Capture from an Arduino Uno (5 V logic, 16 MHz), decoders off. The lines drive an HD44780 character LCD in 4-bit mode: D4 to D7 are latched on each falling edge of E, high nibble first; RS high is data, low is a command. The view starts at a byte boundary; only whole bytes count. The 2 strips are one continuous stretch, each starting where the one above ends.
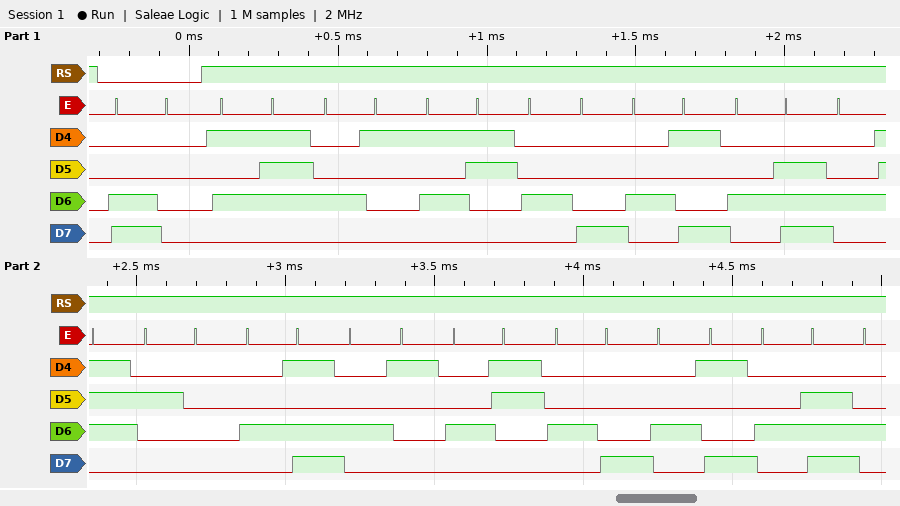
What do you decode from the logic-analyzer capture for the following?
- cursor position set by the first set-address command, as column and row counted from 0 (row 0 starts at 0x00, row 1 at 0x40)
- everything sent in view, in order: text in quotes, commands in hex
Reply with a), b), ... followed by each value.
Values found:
a) column 0, row 1
b) 0xC0 "WASHING MACHIN"
